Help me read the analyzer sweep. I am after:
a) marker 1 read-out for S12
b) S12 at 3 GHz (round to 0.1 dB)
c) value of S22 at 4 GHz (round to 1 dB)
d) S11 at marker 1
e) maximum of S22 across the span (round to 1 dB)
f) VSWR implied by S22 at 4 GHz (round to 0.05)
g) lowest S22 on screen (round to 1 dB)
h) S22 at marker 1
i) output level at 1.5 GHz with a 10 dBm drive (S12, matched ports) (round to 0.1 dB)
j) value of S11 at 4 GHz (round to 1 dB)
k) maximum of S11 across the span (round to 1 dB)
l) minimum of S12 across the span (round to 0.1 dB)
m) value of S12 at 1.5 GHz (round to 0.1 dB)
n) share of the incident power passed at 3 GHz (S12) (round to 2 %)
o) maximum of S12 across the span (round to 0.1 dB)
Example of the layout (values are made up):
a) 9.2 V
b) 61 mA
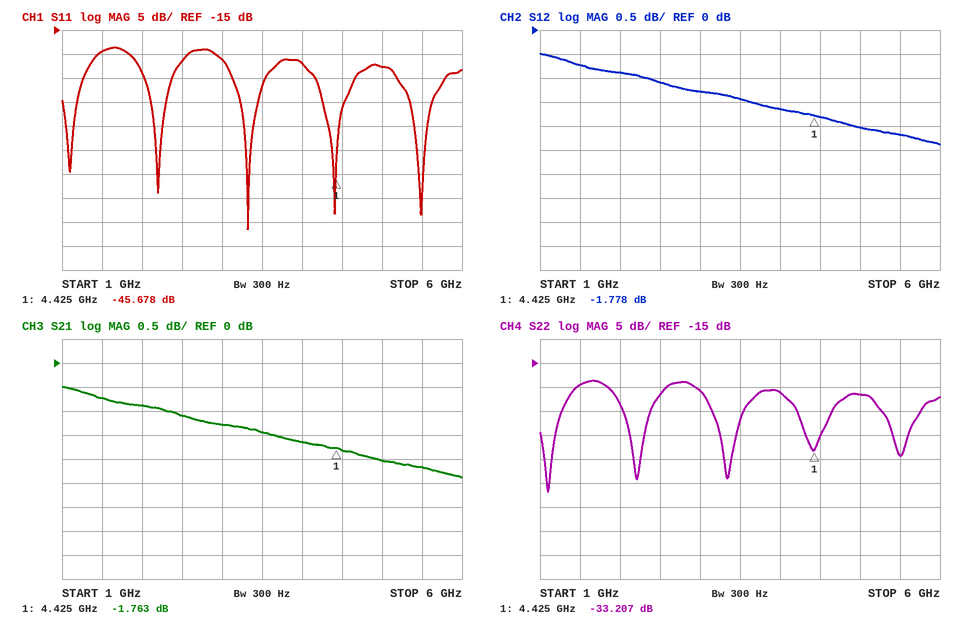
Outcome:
a) -1.778 dB
b) -1.3 dB
c) -21 dB
d) -45.678 dB
e) -19 dB
f) 1.20
g) -42 dB
h) -33.207 dB
i) 9.3 dBm
j) -22 dB
k) -19 dB
l) -2.4 dB
m) -0.7 dB
n) 74 %
o) -0.5 dB
